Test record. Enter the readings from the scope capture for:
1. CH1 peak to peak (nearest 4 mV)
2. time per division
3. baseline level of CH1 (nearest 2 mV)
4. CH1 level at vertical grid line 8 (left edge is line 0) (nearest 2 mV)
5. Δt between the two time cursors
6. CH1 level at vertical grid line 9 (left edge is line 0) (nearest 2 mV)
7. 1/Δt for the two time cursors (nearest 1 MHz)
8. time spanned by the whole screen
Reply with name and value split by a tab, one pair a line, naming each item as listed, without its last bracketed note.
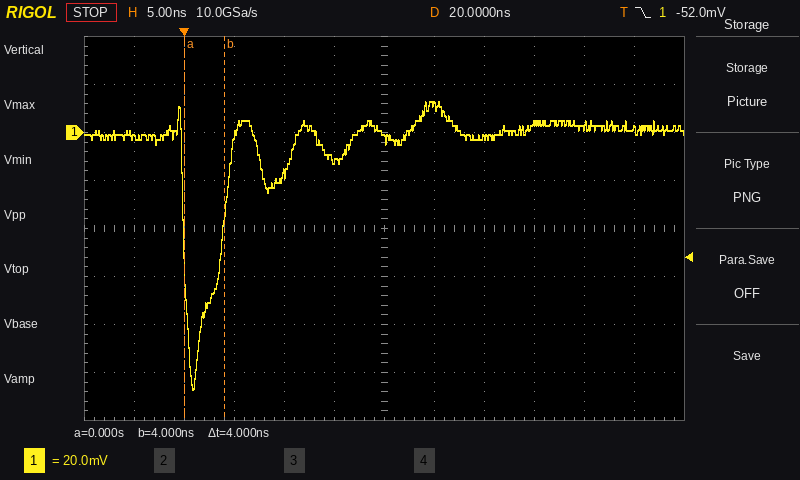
CH1 peak to peak	120 mV
time per division	5 ns
baseline level of CH1	0 mV
CH1 level at vertical grid line 8 (left edge is line 0)	-2 mV
Δt between the two time cursors	4 ns
CH1 level at vertical grid line 9 (left edge is line 0)	4 mV
1/Δt for the two time cursors	250 MHz
time spanned by the whole screen	60 ns
